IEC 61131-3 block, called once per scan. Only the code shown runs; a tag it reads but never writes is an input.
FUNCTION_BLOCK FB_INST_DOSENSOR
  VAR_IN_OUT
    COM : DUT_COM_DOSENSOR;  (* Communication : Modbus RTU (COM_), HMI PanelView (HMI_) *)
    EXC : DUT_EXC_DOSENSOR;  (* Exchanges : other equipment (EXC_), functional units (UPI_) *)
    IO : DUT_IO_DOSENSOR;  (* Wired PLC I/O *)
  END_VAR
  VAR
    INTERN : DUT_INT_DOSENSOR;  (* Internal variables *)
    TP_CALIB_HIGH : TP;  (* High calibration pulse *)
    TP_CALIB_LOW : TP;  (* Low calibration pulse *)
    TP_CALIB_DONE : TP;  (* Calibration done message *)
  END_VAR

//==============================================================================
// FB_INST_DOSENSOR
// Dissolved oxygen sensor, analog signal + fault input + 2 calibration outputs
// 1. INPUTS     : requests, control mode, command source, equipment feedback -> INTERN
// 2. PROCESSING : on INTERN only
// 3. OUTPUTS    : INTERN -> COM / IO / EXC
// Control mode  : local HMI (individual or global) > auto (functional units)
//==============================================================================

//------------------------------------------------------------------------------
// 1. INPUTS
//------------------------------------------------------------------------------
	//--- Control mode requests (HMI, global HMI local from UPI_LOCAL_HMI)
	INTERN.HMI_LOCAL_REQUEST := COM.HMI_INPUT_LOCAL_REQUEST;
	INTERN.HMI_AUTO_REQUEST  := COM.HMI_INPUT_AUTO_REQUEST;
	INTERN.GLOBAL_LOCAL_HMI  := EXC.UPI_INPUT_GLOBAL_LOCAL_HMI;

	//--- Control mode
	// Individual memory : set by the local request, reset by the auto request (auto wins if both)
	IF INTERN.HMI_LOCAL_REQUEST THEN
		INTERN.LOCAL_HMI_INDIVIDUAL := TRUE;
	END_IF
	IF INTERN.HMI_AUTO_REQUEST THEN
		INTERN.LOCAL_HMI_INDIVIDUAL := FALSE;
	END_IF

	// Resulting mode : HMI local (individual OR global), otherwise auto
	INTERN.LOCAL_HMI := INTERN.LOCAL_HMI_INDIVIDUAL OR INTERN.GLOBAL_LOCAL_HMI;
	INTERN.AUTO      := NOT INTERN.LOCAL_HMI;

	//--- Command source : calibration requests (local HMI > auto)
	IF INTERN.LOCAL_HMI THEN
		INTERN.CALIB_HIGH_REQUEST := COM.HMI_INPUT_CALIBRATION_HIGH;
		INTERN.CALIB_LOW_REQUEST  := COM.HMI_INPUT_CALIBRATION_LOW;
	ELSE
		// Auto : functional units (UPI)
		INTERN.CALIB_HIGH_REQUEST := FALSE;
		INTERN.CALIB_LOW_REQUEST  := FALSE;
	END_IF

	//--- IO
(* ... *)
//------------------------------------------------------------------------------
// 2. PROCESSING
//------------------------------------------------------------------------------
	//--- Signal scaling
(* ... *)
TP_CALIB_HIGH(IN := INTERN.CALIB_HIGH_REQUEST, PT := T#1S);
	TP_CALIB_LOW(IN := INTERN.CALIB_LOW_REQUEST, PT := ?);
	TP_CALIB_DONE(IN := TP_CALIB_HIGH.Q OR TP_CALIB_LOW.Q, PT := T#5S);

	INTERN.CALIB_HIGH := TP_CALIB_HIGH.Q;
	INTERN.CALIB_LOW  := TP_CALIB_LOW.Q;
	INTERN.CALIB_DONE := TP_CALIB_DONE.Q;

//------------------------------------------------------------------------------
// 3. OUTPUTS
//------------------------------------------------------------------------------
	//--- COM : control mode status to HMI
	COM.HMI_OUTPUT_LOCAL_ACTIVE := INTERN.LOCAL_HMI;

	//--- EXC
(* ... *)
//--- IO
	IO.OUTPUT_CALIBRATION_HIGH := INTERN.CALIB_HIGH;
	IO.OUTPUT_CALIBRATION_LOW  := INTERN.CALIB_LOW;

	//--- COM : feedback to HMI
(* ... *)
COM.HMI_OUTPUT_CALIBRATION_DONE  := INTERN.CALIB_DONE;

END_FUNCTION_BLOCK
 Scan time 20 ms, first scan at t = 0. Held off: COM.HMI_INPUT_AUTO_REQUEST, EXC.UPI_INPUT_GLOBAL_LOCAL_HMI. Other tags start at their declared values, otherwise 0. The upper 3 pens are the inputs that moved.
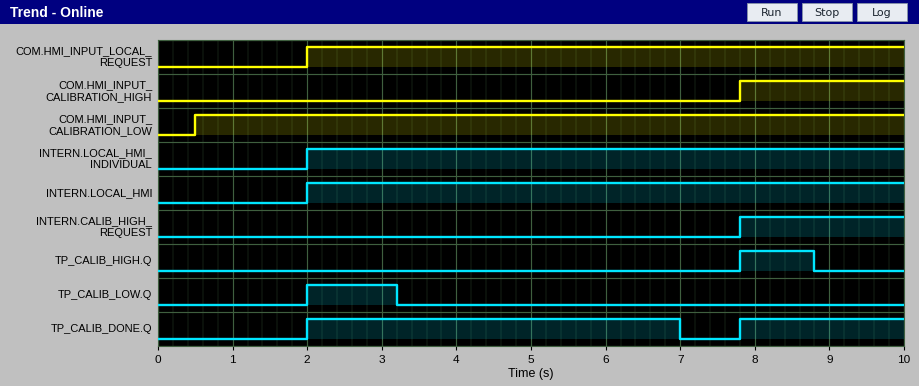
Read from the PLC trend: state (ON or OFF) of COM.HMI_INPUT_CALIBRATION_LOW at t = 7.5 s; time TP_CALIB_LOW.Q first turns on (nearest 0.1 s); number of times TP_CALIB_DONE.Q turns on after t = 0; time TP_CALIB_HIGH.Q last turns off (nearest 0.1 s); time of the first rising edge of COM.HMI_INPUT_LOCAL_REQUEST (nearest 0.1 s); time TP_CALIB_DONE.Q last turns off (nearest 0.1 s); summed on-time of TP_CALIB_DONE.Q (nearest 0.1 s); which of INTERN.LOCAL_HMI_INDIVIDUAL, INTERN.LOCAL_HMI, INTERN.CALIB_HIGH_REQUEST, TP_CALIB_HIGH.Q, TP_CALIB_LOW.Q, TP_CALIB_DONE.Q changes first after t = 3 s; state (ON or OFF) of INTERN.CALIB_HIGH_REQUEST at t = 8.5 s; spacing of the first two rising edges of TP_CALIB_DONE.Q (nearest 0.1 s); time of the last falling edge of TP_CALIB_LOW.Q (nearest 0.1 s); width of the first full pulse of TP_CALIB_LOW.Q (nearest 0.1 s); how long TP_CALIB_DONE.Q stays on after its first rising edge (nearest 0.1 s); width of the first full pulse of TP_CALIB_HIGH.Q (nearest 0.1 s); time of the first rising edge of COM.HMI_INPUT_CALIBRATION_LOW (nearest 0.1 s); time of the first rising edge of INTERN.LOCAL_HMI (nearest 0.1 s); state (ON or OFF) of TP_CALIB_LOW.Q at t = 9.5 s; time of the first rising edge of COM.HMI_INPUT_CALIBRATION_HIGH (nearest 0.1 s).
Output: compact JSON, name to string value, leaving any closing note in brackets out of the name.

{"state (ON or OFF) of COM.HMI_INPUT_CALIBRATION_LOW at t = 7.5 s": "ON", "time TP_CALIB_LOW.Q first turns on": "2.0 s", "number of times TP_CALIB_DONE.Q turns on after t = 0": "2", "time TP_CALIB_HIGH.Q last turns off": "8.8 s", "time of the first rising edge of COM.HMI_INPUT_LOCAL_REQUEST": "2.0 s", "time TP_CALIB_DONE.Q last turns off": "7.0 s", "summed on-time of TP_CALIB_DONE.Q": "7.2 s", "which of INTERN.LOCAL_HMI_INDIVIDUAL, INTERN.LOCAL_HMI, INTERN.CALIB_HIGH_REQUEST, TP_CALIB_HIGH.Q, TP_CALIB_LOW.Q, TP_CALIB_DONE.Q changes first after t = 3 s": "TP_CALIB_LOW.Q", "state (ON or OFF) of INTERN.CALIB_HIGH_REQUEST at t = 8.5 s": "ON", "spacing of the first two rising edges of TP_CALIB_DONE.Q": "5.8 s", "time of the last falling edge of TP_CALIB_LOW.Q": "3.2 s", "width of the first full pulse of TP_CALIB_LOW.Q": "1.2 s", "how long TP_CALIB_DONE.Q stays on after its first rising edge": "5.0 s", "width of the first full pulse of TP_CALIB_HIGH.Q": "1.0 s", "time of the first rising edge of COM.HMI_INPUT_CALIBRATION_LOW": "0.5 s", "time of the first rising edge of INTERN.LOCAL_HMI": "2.0 s", "state (ON or OFF) of TP_CALIB_LOW.Q at t = 9.5 s": "OFF", "time of the first rising edge of COM.HMI_INPUT_CALIBRATION_HIGH": "7.8 s"}
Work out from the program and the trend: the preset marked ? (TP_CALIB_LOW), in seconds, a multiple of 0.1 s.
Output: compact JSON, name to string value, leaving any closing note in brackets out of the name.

{"the preset marked ? (TP_CALIB_LOW), in seconds, a multiple of 0.1 s": "1.2 s"}
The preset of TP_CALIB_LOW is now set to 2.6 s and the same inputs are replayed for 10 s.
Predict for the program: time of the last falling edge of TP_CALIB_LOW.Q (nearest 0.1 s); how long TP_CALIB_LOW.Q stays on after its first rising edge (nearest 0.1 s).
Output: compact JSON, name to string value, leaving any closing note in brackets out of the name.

{"time of the last falling edge of TP_CALIB_LOW.Q": "4.6 s", "how long TP_CALIB_LOW.Q stays on after its first rising edge": "2.6 s"}
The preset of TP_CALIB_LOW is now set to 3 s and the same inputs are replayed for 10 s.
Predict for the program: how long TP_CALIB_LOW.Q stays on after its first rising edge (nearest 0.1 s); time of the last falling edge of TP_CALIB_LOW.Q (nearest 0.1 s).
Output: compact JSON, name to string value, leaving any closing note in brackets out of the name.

{"how long TP_CALIB_LOW.Q stays on after its first rising edge": "3.0 s", "time of the last falling edge of TP_CALIB_LOW.Q": "5.0 s"}
